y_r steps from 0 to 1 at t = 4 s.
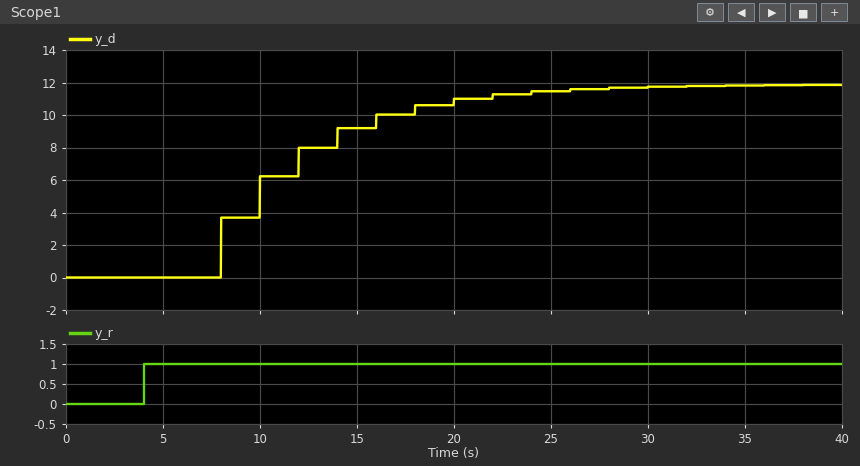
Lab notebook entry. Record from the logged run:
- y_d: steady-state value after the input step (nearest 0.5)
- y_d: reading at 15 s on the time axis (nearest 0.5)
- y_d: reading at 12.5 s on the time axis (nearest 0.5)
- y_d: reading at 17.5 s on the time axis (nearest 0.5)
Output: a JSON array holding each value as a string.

["12.0", "9.0", "8.0", "10.0"]
